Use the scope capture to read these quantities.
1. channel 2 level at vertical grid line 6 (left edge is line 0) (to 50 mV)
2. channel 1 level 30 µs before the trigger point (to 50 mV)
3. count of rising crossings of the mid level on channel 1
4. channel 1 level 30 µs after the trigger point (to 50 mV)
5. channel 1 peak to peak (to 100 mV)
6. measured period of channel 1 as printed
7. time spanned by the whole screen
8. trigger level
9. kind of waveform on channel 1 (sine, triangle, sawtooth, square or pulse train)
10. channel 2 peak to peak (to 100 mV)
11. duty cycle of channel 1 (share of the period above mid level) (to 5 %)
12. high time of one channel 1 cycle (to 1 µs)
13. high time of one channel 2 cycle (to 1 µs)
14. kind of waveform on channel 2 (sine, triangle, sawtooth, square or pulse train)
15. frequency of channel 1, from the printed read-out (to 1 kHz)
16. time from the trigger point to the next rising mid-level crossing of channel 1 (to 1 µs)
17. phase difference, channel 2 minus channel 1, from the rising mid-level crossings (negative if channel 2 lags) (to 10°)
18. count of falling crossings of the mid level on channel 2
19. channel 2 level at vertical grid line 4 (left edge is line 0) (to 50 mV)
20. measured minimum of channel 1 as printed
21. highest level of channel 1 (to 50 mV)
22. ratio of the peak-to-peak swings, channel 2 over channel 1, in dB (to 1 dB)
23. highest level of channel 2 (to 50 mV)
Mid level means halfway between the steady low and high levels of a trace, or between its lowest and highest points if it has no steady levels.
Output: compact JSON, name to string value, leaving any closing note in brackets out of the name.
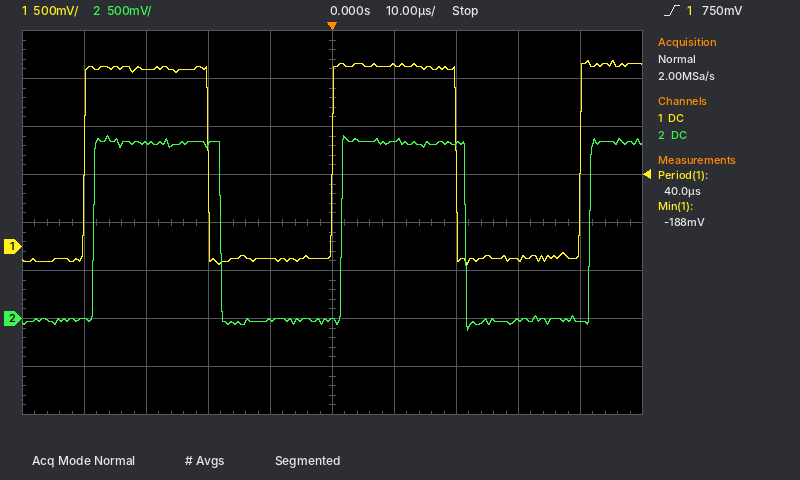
{"channel 2 level at vertical grid line 6 (left edge is line 0)": "1.85 V", "channel 1 level 30 µs before the trigger point": "1.85 V", "count of rising crossings of the mid level on channel 1": "3", "channel 1 level 30 µs after the trigger point": "-150 mV", "channel 1 peak to peak": "2.10 V", "measured period of channel 1 as printed": "40.0 µs", "time spanned by the whole screen": "100 µs", "trigger level": "750 mV", "kind of waveform on channel 1": "square", "channel 2 peak to peak": "2.00 V", "duty cycle of channel 1 (share of the period above mid level)": "50 %", "high time of one channel 1 cycle": "20 µs", "high time of one channel 2 cycle": "20 µs", "kind of waveform on channel 2": "square", "frequency of channel 1, from the printed read-out": "25 kHz", "time from the trigger point to the next rising mid-level crossing of channel 1": "40 µs", "phase difference, channel 2 minus channel 1, from the rising mid-level crossings (negative if channel 2 lags)": "-10°", "count of falling crossings of the mid level on channel 2": "2", "channel 2 level at vertical grid line 4 (left edge is line 0)": "0 mV", "measured minimum of channel 1 as printed": "-188 mV", "highest level of channel 1": "1.95 V", "ratio of the peak-to-peak swings, channel 2 over channel 1, in dB": "0 dB", "highest level of channel 2": "1.90 V"}
